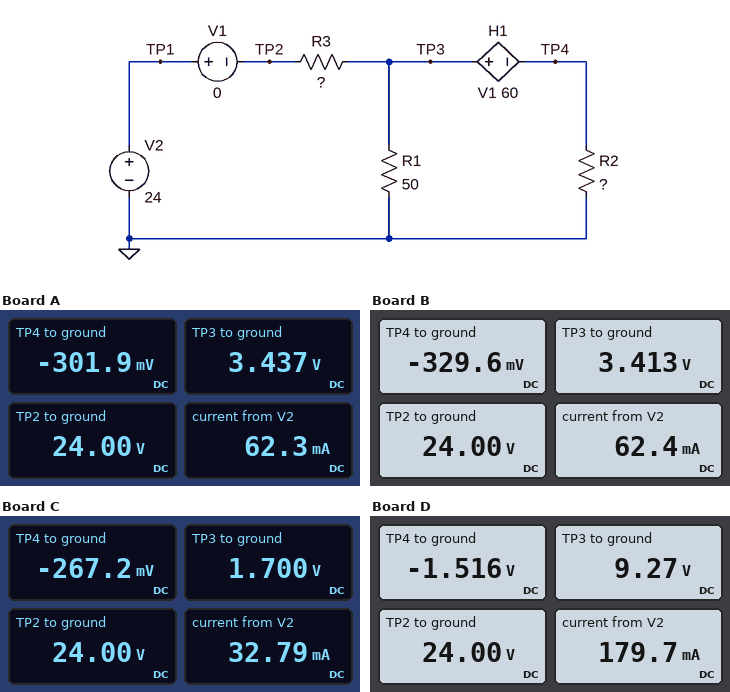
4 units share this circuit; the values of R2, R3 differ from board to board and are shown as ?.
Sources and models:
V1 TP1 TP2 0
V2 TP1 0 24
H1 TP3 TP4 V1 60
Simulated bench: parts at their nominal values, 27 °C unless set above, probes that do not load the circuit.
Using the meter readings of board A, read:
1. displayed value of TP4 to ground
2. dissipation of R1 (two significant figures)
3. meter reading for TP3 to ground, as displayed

-301.9 mV
240 mW
3.437 V
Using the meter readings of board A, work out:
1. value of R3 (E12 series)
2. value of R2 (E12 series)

330 Ω
47 Ω
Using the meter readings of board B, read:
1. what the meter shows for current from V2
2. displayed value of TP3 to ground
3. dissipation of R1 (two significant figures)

62.4 mA
3.413 V
230 mW
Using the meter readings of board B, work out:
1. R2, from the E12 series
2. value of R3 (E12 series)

56 Ω
330 Ω
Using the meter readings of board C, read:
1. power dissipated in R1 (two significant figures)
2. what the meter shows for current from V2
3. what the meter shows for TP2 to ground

58 mW
32.79 mA
24.00 V
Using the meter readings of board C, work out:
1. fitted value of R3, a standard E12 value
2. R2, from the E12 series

680 Ω
220 Ω
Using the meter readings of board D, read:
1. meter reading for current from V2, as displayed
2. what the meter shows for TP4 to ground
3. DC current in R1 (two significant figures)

179.7 mA
-1.516 V
190 mA
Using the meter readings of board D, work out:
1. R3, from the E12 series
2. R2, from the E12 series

82 Ω
270 Ω
